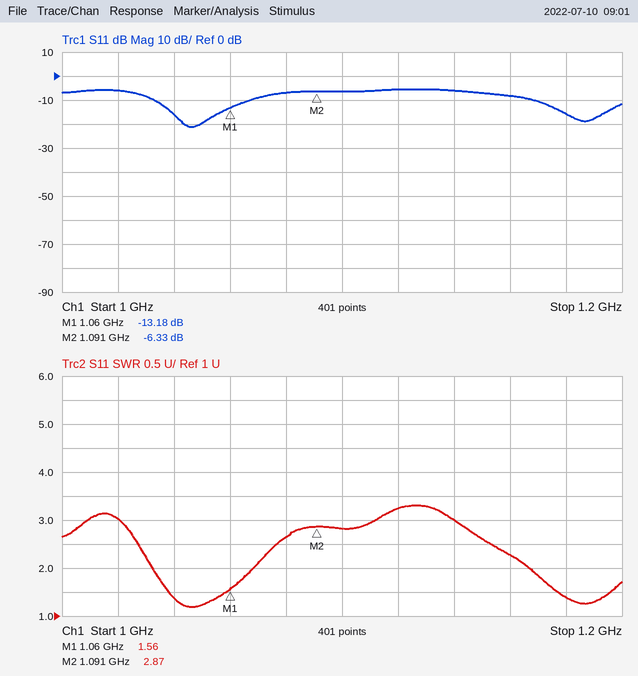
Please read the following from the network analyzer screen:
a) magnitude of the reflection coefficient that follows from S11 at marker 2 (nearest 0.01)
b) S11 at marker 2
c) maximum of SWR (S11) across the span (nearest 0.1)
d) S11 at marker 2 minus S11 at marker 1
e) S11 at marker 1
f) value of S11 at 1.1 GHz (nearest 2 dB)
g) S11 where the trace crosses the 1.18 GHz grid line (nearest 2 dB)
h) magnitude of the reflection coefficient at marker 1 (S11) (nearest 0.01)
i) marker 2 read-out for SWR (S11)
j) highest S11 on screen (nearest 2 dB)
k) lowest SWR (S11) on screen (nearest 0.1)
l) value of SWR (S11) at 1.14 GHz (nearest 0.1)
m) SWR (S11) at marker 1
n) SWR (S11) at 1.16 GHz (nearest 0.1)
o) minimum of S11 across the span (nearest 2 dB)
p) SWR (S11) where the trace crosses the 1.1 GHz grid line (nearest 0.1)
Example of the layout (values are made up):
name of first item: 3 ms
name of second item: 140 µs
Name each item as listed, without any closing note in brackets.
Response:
magnitude of the reflection coefficient that follows from S11 at marker 2: 0.48
S11 at marker 2: -6.33 dB
maximum of SWR (S11) across the span: 3.3
S11 at marker 2 minus S11 at marker 1: 6.85 dB
S11 at marker 1: -13.18 dB
value of S11 at 1.1 GHz: -6 dB
S11 where the trace crosses the 1.18 GHz grid line: -16 dB
magnitude of the reflection coefficient at marker 1 (S11): 0.22
marker 2 read-out for SWR: 2.87
highest S11 on screen: -6 dB
lowest SWR (S11) on screen: 1.2
value of SWR (S11) at 1.14 GHz: 3.0
SWR (S11) at marker 1: 1.56
SWR (S11) at 1.16 GHz: 2.3
minimum of S11 across the span: -22 dB
SWR (S11) where the trace crosses the 1.1 GHz grid line: 2.8
